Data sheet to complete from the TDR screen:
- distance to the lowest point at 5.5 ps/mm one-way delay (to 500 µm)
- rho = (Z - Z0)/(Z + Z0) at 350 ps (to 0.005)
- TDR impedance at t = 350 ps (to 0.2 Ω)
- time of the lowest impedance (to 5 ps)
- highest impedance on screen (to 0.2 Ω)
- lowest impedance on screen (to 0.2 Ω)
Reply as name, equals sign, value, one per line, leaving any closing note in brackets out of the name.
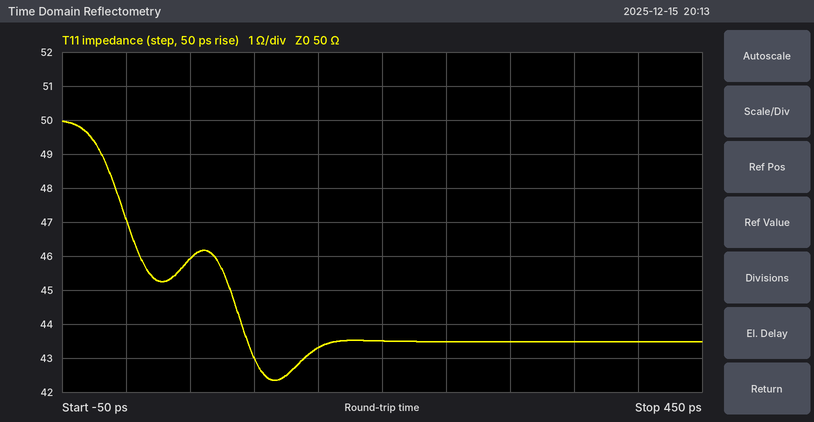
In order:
distance to the lowest point at 5.5 ps/mm one-way delay = 10.5 mm
rho = (Z - Z0)/(Z + Z0) at 350 ps = -0.070
TDR impedance at t = 350 ps = 43.4 Ω
time of the lowest impedance = 115 ps
highest impedance on screen = 50.0 Ω
lowest impedance on screen = 42.4 Ω
